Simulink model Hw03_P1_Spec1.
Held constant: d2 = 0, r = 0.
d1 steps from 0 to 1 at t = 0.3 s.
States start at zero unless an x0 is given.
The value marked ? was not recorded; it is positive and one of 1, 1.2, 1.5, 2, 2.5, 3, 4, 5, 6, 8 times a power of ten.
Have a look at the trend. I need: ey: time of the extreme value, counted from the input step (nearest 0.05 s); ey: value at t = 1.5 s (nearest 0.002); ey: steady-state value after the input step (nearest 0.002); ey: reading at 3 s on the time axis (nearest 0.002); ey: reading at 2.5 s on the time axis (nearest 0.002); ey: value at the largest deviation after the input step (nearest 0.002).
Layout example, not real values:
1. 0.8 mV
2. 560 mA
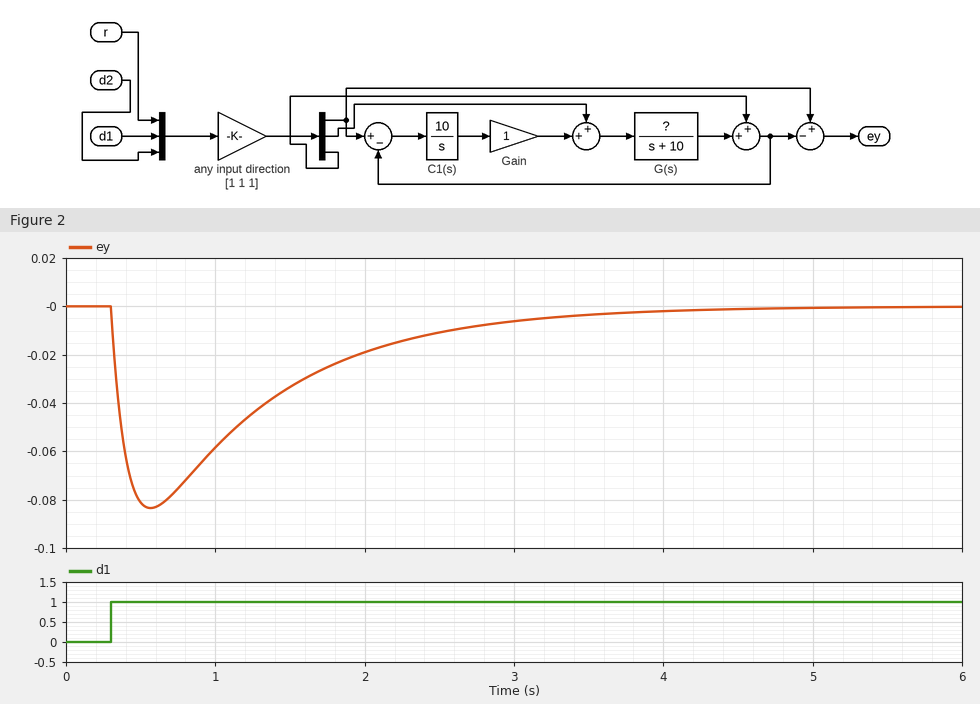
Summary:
1. 0.25 s
2. -0.034
3. 0.000
4. -0.006
5. -0.010
6. -0.084
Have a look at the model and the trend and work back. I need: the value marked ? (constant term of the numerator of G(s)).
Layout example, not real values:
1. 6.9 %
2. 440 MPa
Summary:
1. 1
